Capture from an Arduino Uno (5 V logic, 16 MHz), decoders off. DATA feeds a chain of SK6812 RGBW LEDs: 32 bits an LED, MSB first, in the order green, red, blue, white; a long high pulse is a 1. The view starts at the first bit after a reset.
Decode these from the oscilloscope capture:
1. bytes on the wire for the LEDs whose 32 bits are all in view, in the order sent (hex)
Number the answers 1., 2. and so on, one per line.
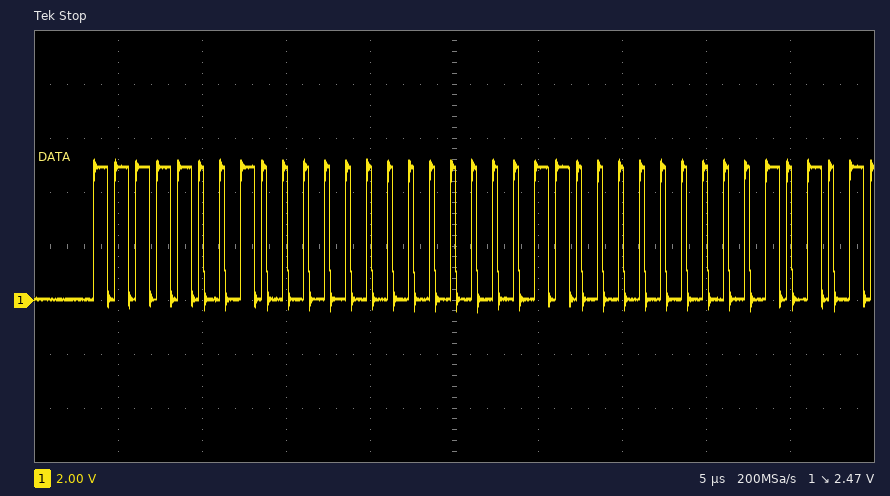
1. F9 00 06 00
